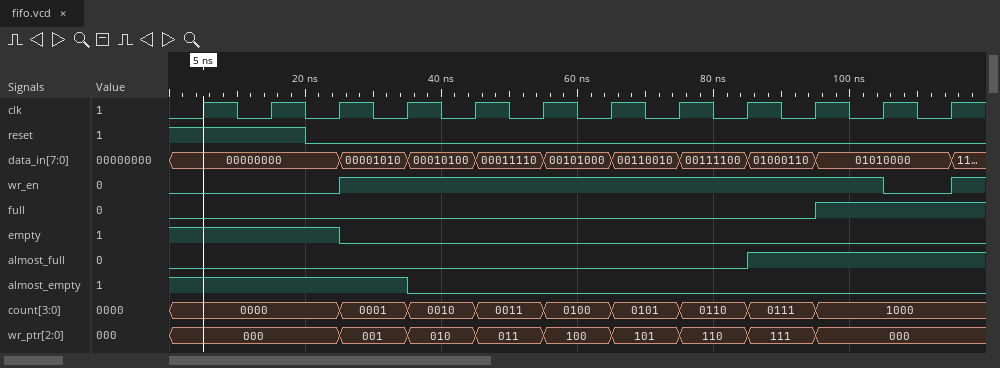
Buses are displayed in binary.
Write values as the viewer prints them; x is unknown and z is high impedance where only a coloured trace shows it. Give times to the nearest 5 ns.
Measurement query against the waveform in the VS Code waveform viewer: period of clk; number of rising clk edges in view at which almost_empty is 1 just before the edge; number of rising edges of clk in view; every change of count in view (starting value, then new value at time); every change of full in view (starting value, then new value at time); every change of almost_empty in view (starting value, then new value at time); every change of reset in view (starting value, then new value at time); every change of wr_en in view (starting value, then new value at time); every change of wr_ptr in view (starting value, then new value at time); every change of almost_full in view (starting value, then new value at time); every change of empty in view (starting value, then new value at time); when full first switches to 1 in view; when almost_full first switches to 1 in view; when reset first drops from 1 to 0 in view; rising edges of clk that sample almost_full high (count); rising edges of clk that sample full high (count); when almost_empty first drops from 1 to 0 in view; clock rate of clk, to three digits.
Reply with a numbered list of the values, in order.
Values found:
1. 10 ns
2. 4
3. 12
4. 0000, 0001 at 25 ns, 0010 at 35 ns, 0011 at 45 ns, 0100 at 55 ns, 0101 at 65 ns, 0110 at 75 ns, 0111 at 85 ns, 1000 at 95 ns
5. 0, 1 at 95 ns
6. 1, 0 at 35 ns
7. 1, 0 at 20 ns
8. 0, 1 at 25 ns, 0 at 105 ns, 1 at 115 ns
9. 000, 001 at 25 ns, 010 at 35 ns, 011 at 45 ns, 100 at 55 ns, 101 at 65 ns, 110 at 75 ns, 111 at 85 ns, 000 at 95 ns
10. 0, 1 at 85 ns
11. 1, 0 at 25 ns
12. 95 ns
13. 85 ns
14. 20 ns
15. 3
16. 2
17. 35 ns
18. 100 MHz
